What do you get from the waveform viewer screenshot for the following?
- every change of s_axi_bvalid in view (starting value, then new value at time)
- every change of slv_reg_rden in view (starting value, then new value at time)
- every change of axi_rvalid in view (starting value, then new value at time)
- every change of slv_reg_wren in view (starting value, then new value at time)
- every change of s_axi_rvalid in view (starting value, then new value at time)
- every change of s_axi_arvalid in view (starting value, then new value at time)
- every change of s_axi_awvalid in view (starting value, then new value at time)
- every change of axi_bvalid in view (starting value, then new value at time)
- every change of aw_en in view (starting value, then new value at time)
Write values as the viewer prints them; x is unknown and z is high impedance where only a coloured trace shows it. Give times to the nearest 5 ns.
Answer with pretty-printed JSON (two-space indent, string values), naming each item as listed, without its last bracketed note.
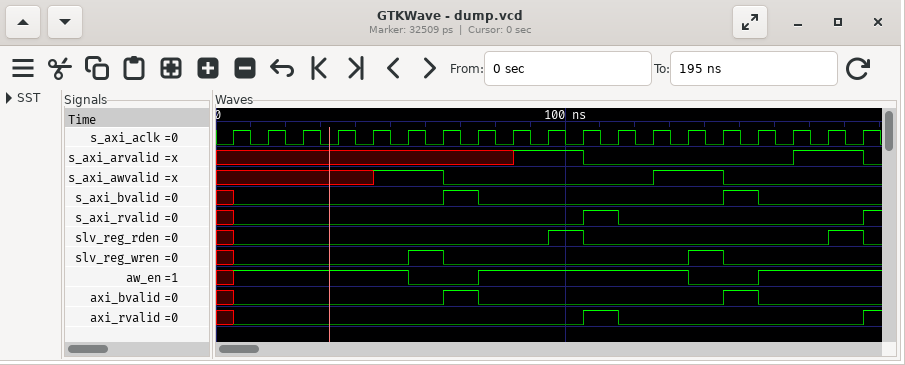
{
  "every change of s_axi_bvalid in view": "x, 0 at 5 ns, 1 at 65 ns, 0 at 75 ns, 1 at 145 ns, 0 at 155 ns",
  "every change of slv_reg_rden in view": "x, 0 at 5 ns, 1 at 95 ns, 0 at 105 ns, 1 at 175 ns, 0 at 185 ns",
  "every change of axi_rvalid in view": "x, 0 at 5 ns, 1 at 105 ns, 0 at 115 ns, 1 at 185 ns",
  "every change of slv_reg_wren in view": "x, 0 at 5 ns, 1 at 55 ns, 0 at 65 ns, 1 at 135 ns, 0 at 145 ns",
  "every change of s_axi_rvalid in view": "x, 0 at 5 ns, 1 at 105 ns, 0 at 115 ns, 1 at 185 ns",
  "every change of s_axi_arvalid in view": "x, 1 at 85 ns, 0 at 105 ns, 1 at 165 ns, 0 at 185 ns",
  "every change of s_axi_awvalid in view": "x, 1 at 45 ns, 0 at 65 ns, 1 at 125 ns, 0 at 145 ns",
  "every change of axi_bvalid in view": "x, 0 at 5 ns, 1 at 65 ns, 0 at 75 ns, 1 at 145 ns, 0 at 155 ns",
  "every change of aw_en in view": "x, 1 at 5 ns, 0 at 55 ns, 1 at 75 ns, 0 at 135 ns, 1 at 155 ns"
}
